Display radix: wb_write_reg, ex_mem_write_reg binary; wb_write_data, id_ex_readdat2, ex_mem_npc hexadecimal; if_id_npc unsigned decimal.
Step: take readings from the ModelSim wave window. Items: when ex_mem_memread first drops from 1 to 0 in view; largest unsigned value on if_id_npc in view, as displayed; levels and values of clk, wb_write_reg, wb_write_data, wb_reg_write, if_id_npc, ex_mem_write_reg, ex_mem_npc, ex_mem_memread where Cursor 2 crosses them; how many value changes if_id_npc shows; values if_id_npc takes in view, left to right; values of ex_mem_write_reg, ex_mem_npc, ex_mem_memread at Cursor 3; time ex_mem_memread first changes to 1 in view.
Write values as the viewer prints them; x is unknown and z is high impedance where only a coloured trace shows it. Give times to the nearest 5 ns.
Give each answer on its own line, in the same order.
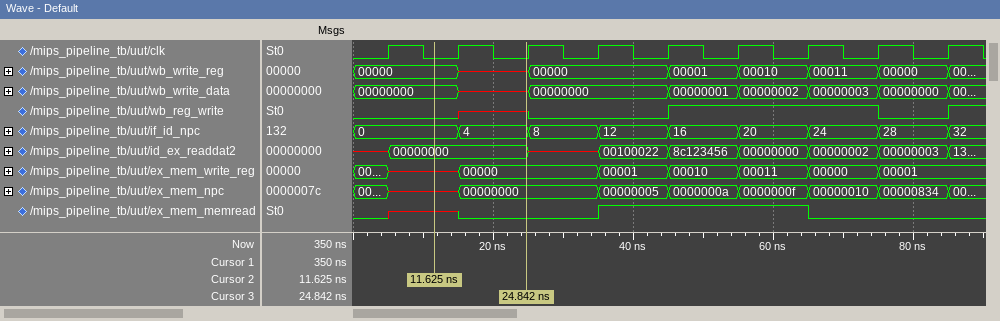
65 ns
32
clk=0, wb_write_reg=00000, wb_write_data=00000000, wb_reg_write=0, if_id_npc=0, ex_mem_write_reg=x, ex_mem_npc=x, ex_mem_memread=x
8
0, 4, 8, 12, 16, 20, 24, 28, 32
ex_mem_write_reg=00000, ex_mem_npc=00000000, ex_mem_memread=0
35 ns
